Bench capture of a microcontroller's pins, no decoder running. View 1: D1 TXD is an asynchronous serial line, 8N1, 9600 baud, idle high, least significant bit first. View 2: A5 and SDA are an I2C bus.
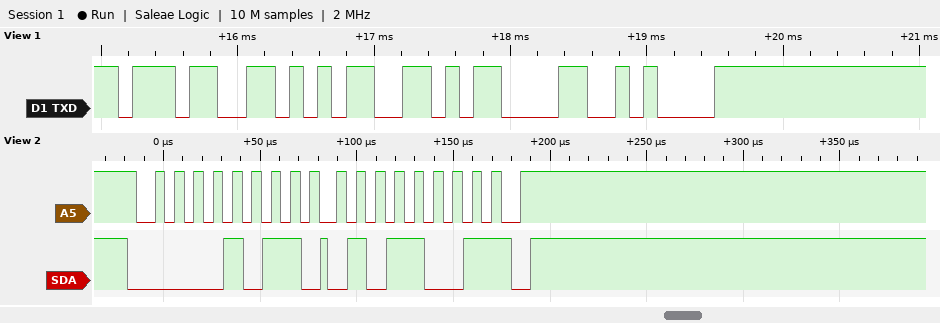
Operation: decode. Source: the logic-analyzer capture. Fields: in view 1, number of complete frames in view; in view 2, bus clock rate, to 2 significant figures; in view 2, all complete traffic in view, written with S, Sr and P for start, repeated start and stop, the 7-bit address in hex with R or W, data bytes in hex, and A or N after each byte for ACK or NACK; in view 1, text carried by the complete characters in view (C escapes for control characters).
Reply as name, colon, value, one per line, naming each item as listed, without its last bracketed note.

in view 1, number of complete frames in view: 4
in view 2, bus clock rate, to 2 significant figures: 100 kHz
in view 2, all complete traffic in view, written with S, Sr and P for start, repeated start and stop, the 7-bit address in hex with R or W, data bytes in hex, and A or N after each byte for ACK or NACK: S 05R A 59 N P
in view 1, text carried by the complete characters in view: "75\r\n"
